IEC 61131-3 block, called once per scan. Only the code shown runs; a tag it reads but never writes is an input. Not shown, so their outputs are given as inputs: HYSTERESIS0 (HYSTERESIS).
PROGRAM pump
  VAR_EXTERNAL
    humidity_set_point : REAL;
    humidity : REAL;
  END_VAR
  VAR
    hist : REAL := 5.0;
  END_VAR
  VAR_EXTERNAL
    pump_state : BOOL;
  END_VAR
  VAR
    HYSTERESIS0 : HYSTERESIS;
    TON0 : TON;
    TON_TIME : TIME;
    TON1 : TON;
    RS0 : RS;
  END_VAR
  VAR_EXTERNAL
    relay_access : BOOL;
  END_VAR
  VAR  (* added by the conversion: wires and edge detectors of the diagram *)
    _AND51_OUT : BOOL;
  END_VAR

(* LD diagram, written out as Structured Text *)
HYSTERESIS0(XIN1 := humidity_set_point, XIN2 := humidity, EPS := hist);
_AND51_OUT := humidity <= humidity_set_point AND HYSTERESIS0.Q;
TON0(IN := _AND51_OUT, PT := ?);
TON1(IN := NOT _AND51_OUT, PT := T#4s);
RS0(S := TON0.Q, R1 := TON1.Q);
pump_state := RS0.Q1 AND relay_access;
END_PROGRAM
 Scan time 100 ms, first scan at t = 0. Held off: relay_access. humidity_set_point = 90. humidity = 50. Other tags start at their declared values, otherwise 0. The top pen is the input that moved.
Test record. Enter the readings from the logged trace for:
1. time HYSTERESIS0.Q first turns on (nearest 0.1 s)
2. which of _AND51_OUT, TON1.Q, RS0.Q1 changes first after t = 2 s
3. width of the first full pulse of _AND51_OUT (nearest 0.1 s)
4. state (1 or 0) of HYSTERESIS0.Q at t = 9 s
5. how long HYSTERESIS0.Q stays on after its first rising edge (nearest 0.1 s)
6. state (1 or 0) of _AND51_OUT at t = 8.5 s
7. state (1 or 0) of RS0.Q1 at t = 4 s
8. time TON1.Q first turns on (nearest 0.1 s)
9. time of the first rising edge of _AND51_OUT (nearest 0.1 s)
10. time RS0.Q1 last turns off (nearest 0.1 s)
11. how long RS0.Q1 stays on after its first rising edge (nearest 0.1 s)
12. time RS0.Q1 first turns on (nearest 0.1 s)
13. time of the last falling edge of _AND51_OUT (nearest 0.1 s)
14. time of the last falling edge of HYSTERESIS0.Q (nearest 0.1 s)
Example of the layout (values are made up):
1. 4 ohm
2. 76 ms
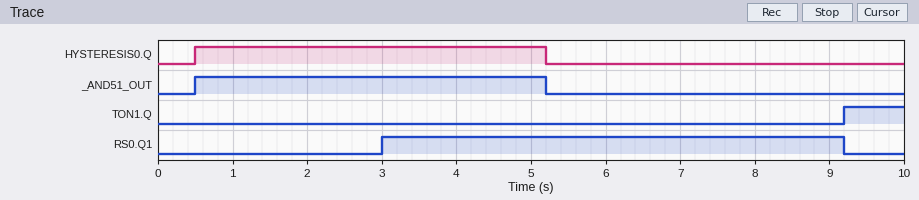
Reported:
1. 0.5 s
2. RS0.Q1
3. 4.7 s
4. 0
5. 4.7 s
6. 0
7. 1
8. 9.2 s
9. 0.5 s
10. 9.2 s
11. 6.2 s
12. 3.0 s
13. 5.2 s
14. 5.2 s
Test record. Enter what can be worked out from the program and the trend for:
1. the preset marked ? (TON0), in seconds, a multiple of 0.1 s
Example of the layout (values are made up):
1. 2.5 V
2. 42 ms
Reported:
1. 2.5 s
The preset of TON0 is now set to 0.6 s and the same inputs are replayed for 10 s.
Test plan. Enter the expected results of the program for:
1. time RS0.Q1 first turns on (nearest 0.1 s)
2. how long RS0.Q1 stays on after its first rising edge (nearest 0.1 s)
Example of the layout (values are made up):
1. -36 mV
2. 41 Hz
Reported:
1. 1.1 s
2. 8.1 s
